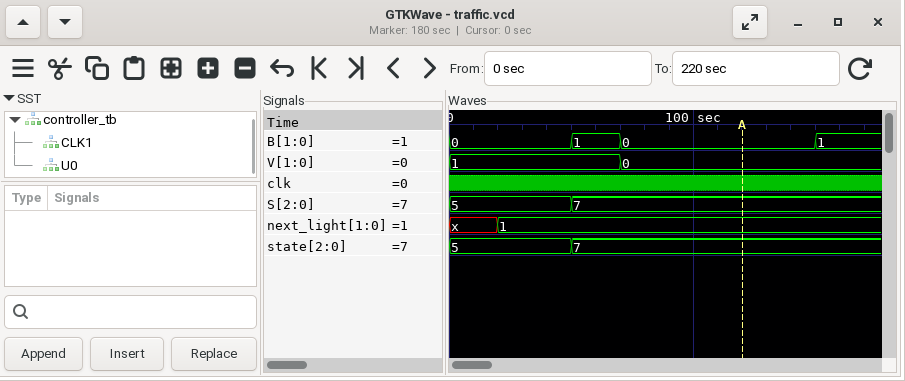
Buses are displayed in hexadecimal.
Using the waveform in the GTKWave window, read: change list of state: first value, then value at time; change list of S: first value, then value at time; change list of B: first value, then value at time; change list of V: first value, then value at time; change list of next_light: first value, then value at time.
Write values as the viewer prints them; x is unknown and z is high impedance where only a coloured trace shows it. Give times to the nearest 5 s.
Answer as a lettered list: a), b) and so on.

a) 5, 7 at 50 s
b) 5, 7 at 50 s
c) 0, 1 at 50 s, 0 at 70 s, 1 at 150 s
d) 1, 0 at 70 s
e) x, 1 at 20 s
